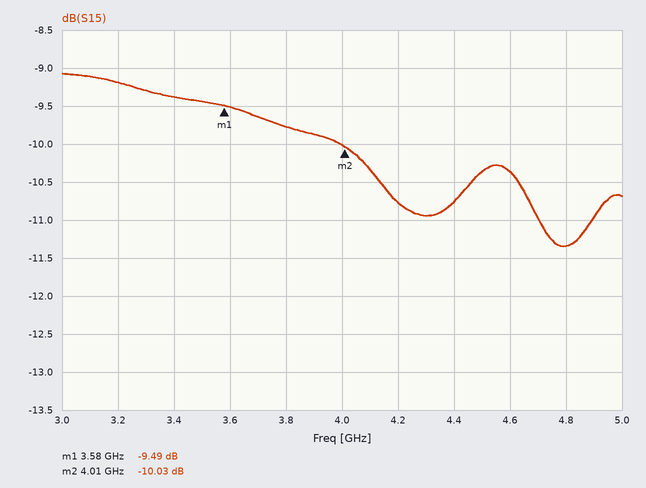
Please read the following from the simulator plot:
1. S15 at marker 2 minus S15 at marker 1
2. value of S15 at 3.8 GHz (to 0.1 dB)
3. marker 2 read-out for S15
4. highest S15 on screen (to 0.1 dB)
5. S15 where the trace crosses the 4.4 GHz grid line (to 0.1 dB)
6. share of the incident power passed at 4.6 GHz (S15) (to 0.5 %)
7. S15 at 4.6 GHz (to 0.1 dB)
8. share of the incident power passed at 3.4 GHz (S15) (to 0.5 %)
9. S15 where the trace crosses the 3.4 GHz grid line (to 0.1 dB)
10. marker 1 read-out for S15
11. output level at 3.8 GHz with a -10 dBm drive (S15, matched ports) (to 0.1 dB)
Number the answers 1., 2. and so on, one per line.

1. -0.54 dB
2. -9.8 dB
3. -10.03 dB
4. -9.1 dB
5. -10.8 dB
6. 9.0 %
7. -10.4 dB
8. 11.5 %
9. -9.4 dB
10. -9.49 dB
11. -19.8 dBm
